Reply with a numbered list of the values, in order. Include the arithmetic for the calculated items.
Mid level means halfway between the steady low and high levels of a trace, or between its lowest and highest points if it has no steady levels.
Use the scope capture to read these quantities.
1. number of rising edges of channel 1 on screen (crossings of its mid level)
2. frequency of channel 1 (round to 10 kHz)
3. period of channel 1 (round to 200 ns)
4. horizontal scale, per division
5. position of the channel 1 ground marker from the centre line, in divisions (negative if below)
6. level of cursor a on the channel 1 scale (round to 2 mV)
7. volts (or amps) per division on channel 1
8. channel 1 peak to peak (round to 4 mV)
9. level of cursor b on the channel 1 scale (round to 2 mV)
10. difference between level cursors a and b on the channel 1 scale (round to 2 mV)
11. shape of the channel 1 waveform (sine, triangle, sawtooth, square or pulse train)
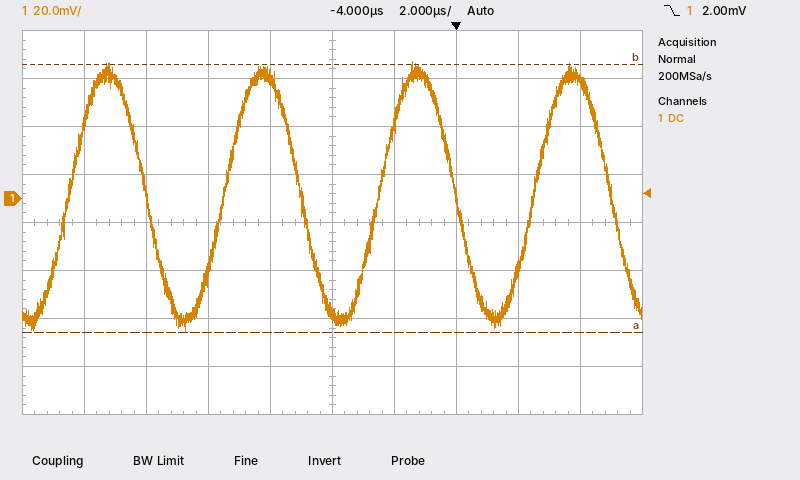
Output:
1. 4
2. 1 / 5.0 µs ≈ 200 kHz
3. 5.0 µs
4. 2 µs
5. +0.5 div
6. -56 mV
7. 20 mV
8. 112 mV
9. 56 mV
10. 112 mV
11. sine
